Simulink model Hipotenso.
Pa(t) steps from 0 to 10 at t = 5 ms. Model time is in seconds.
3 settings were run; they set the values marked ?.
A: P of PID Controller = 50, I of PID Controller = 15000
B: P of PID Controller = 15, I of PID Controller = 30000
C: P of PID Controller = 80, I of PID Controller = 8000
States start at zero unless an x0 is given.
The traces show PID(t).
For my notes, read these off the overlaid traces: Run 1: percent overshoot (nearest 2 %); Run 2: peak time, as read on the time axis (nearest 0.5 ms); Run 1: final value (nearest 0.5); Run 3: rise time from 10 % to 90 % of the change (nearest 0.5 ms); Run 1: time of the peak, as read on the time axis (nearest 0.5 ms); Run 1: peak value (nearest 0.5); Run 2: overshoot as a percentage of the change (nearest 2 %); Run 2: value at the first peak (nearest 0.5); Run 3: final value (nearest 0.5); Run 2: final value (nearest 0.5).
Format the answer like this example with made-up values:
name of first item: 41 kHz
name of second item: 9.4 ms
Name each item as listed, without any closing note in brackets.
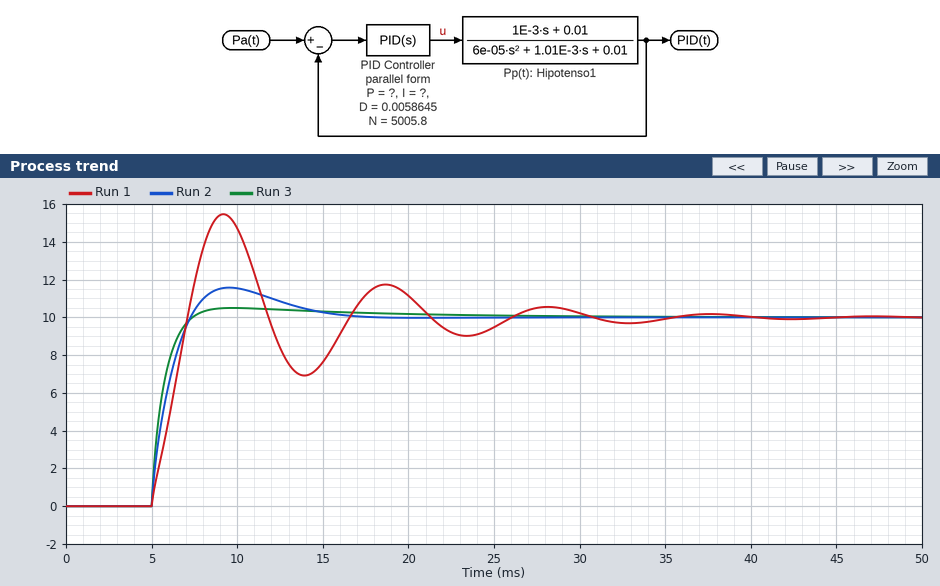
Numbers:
Run 1: percent overshoot: 54 %
Run 2: peak time, as read on the time axis: 9.5 ms
Run 1: final value: 10.0
Run 3: rise time from 10 % to 90 % of the change: 1.5 ms
Run 1: time of the peak, as read on the time axis: 9.0 ms
Run 1: peak value: 15.5
Run 2: overshoot as a percentage of the change: 16 %
Run 2: value at the first peak: 11.5
Run 3: final value: 10.0
Run 2: final value: 10.0
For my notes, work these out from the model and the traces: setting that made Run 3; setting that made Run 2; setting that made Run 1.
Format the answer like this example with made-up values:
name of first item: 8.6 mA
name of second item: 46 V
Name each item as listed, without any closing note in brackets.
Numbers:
setting that made Run 3: C
setting that made Run 2: A
setting that made Run 1: B
